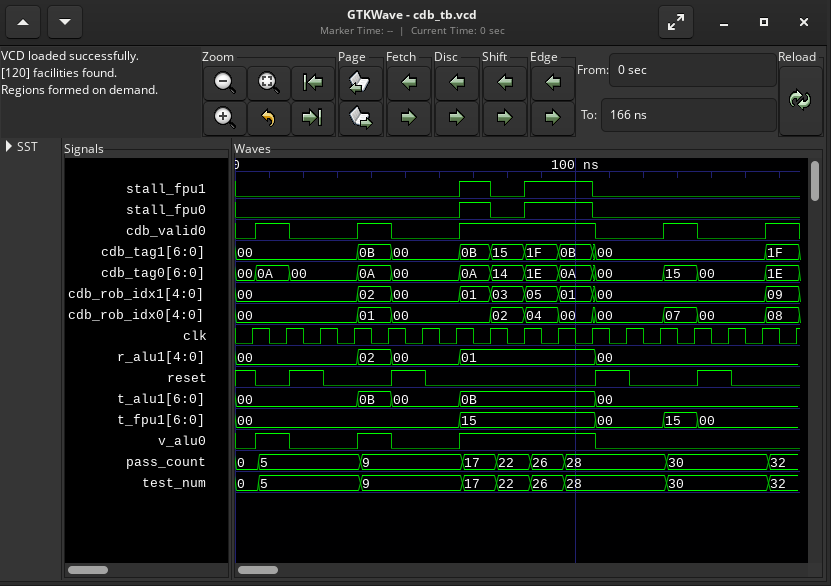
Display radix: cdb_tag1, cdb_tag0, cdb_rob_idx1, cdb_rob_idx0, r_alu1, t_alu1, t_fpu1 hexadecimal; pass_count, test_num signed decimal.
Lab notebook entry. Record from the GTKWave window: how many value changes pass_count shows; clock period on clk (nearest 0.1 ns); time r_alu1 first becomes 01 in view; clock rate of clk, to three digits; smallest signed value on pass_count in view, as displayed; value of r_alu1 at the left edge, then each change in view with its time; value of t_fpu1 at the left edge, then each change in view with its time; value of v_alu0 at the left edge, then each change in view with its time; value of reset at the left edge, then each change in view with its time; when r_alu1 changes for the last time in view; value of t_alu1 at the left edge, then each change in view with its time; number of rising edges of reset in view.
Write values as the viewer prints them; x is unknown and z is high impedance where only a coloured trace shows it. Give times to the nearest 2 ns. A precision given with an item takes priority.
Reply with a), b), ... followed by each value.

a) 8
b) 10 ns
c) 66 ns
d) 100 MHz
e) 0
f) 00, 02 at 36 ns, 00 at 46 ns, 01 at 66 ns, 00 at 106 ns
g) 00, 15 at 66 ns, 00 at 106 ns, 15 at 126 ns, 00 at 136 ns
h) 0, 1 at 6 ns, 0 at 16 ns, 1 at 36 ns, 0 at 46 ns, 1 at 66 ns, 0 at 106 ns
i) 1, 0 at 6 ns, 1 at 16 ns, 0 at 26 ns, 1 at 46 ns, 0 at 56 ns, 1 at 106 ns, 0 at 116 ns, 1 at 136 ns, 0 at 146 ns
j) 106 ns
k) 00, 0B at 36 ns, 00 at 46 ns, 0B at 66 ns, 00 at 106 ns
l) 4
